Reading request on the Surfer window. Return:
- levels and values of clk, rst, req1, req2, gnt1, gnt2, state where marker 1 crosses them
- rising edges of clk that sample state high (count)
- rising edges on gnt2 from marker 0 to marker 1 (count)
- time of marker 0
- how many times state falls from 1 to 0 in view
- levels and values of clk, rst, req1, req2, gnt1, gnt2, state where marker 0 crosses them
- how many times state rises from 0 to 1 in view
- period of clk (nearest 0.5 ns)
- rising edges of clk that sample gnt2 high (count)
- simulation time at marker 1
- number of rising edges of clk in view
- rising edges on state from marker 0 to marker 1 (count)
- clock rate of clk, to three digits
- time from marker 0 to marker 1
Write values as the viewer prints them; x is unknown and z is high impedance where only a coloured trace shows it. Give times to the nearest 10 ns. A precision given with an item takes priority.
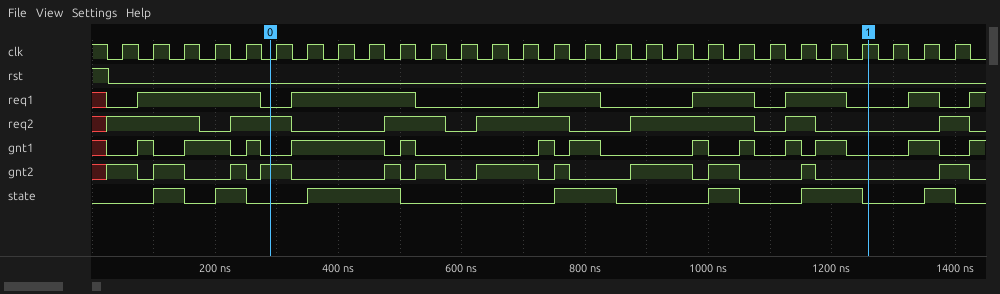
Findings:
clk=1, rst=0, req1=0, req2=0, gnt1=0, gnt2=0, state=0
11
7
290 ns
7
clk=0, rst=0, req1=0, req2=1, gnt1=0, gnt2=1, state=0
7
50 ns
12
1260 ns
28
4
20.0 MHz
970 ns
